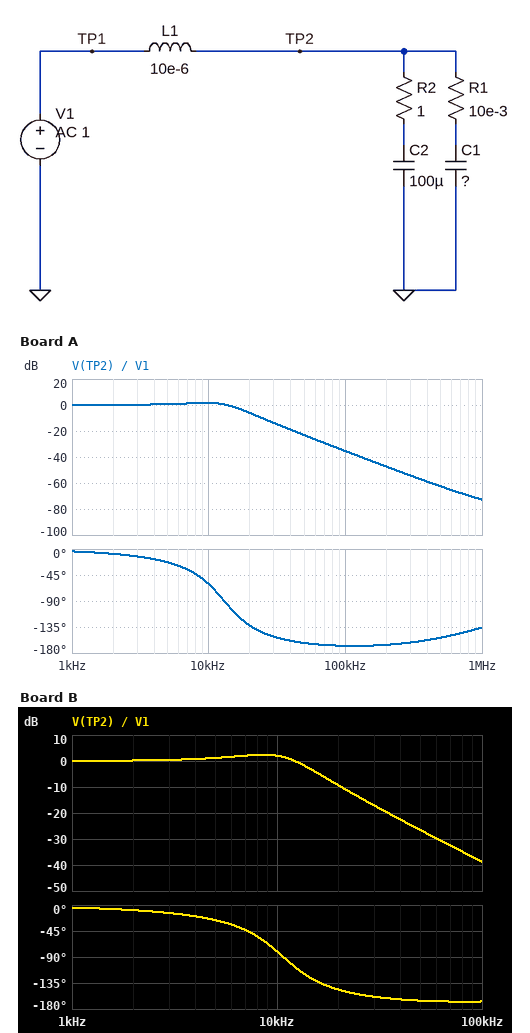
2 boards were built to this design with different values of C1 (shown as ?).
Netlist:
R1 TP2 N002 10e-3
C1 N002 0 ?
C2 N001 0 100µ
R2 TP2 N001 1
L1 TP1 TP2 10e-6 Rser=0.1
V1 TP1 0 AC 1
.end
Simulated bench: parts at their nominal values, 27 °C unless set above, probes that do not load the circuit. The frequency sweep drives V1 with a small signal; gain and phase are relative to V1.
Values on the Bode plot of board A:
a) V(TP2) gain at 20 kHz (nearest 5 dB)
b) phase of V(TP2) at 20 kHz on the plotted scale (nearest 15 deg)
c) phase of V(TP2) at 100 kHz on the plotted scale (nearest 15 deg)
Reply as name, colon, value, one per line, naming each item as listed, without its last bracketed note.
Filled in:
V(TP2) gain at 20 kHz: -5 dB
phase of V(TP2) at 20 kHz on the plotted scale: -135 deg
phase of V(TP2) at 100 kHz on the plotted scale: -165 deg
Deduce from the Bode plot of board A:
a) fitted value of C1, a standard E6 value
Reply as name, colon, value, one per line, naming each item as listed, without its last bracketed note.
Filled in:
fitted value of C1, a standard E6 value: 15 µF
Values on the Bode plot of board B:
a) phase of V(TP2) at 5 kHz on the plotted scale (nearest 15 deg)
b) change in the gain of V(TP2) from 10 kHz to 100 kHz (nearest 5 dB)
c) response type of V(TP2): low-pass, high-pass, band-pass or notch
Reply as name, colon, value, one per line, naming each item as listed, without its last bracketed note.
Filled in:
phase of V(TP2) at 5 kHz on the plotted scale: -30 deg
change in the gain of V(TP2) from 10 kHz to 100 kHz: -40 dB
response type of V(TP2): low-pass, high-pass, band-pass or notch: low-pass
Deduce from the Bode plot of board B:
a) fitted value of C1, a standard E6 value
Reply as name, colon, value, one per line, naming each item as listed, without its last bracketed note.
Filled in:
fitted value of C1, a standard E6 value: 22 µF
